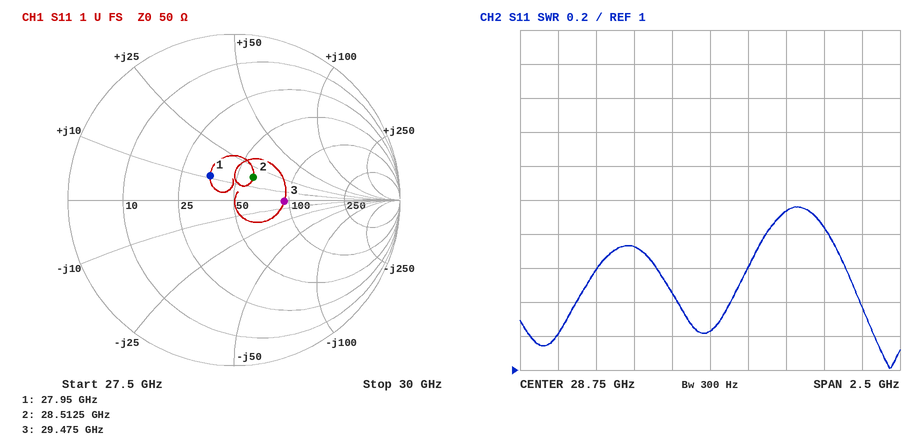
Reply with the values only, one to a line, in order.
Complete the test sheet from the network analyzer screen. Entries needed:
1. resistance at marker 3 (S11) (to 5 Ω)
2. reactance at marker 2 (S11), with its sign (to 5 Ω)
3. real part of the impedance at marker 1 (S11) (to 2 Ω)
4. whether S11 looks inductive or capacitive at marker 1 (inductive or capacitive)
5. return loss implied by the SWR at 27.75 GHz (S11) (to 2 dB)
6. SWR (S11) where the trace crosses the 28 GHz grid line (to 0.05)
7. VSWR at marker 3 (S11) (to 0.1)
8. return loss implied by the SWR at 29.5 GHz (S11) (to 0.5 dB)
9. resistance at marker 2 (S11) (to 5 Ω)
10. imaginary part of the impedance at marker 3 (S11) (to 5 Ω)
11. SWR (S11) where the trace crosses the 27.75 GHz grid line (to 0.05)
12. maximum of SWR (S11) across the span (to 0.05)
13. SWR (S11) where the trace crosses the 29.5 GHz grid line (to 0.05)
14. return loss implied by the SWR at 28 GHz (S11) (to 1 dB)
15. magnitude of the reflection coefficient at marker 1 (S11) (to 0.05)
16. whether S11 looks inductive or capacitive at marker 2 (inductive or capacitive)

95 Ω
+15 Ω
36 Ω
inductive
20 dB
1.60
1.9
10.5 dB
60 Ω
0 Ω
1.20
1.95
1.85
13 dB
0.20
inductive
